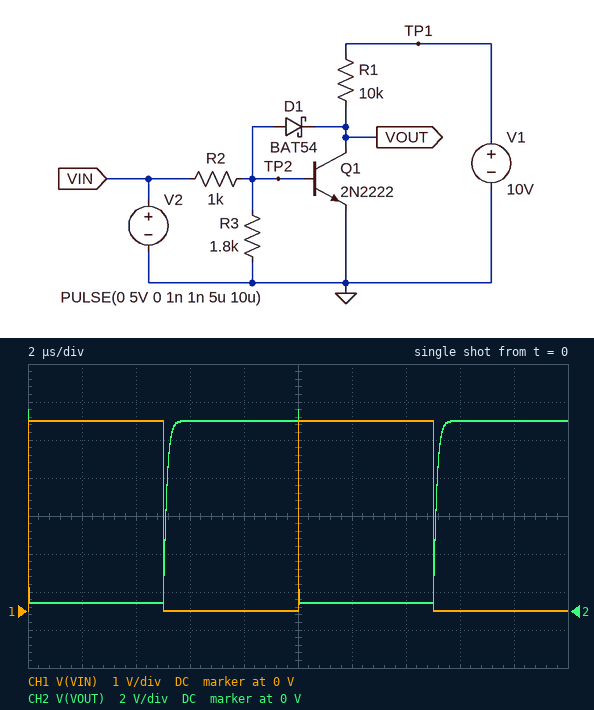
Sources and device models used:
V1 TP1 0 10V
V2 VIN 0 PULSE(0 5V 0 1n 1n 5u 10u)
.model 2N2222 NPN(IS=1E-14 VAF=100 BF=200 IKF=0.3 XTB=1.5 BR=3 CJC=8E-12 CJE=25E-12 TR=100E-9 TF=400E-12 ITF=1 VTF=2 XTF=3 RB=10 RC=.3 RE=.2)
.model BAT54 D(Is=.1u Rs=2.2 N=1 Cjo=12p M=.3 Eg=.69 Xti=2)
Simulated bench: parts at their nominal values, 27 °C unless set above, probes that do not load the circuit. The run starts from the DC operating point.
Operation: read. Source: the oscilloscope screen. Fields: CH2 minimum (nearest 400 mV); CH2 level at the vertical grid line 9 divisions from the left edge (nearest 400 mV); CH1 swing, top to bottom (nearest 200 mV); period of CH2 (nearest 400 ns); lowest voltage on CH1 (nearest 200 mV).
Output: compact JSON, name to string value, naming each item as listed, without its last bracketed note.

{"CH2 minimum": "400 mV", "CH2 level at the vertical grid line 9 divisions from the left edge": "10.0 V", "CH1 swing, top to bottom": "5.0 V", "period of CH2": "10.0 µs", "lowest voltage on CH1": "0 V"}
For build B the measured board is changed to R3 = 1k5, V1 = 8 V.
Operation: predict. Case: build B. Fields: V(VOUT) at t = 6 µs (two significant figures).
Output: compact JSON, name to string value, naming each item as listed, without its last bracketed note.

{"V(VOUT) at t = 6 µs": "8.0 V"}
